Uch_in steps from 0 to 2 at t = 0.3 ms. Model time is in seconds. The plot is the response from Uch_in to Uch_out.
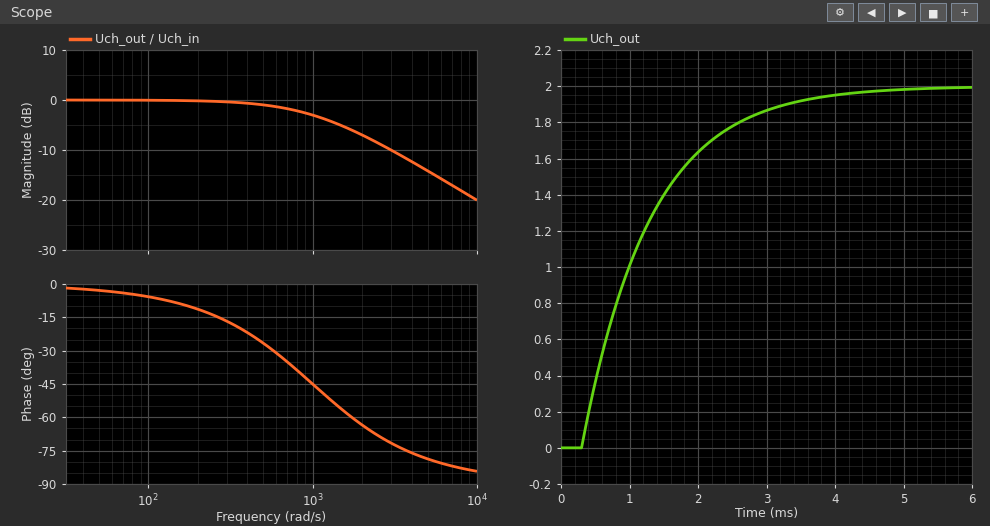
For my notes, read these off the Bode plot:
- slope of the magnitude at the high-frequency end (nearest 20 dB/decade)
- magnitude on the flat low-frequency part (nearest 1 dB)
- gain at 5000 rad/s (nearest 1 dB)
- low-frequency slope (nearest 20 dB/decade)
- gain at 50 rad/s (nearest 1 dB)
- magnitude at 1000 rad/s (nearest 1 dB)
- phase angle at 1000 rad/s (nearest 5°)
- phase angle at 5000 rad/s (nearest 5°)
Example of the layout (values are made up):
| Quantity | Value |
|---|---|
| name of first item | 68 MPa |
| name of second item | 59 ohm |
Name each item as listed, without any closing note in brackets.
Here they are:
| Quantity | Value |
|---|---|
| slope of the magnitude at the high-frequency end | -20 dB/decade |
| magnitude on the flat low-frequency part | 0 dB |
| gain at 5000 rad/s | -14 dB |
| low-frequency slope | 0 dB/decade |
| gain at 50 rad/s | 0 dB |
| magnitude at 1000 rad/s | -3 dB |
| phase angle at 1000 rad/s | -45° |
| phase angle at 5000 rad/s | -80° |
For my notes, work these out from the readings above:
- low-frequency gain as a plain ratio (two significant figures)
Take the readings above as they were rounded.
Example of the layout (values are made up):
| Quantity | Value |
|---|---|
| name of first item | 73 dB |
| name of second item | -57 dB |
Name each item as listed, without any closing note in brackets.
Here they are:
| Quantity | Value |
|---|---|
| low-frequency gain as a plain ratio | 1.0 |
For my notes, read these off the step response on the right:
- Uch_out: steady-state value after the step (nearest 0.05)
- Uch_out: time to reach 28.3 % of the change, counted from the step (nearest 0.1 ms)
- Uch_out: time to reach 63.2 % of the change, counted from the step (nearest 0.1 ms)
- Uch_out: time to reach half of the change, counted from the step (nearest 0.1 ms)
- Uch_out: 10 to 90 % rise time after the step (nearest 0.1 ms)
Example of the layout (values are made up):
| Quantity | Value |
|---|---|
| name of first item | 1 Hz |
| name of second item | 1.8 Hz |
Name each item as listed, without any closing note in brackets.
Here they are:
| Quantity | Value |
|---|---|
| Uch_out: steady-state value after the step | 2.00 |
| Uch_out: time to reach 28.3 % of the change, counted from the step | 0.3 ms |
| Uch_out: time to reach 63.2 % of the change, counted from the step | 1.0 ms |
| Uch_out: time to reach half of the change, counted from the step | 0.7 ms |
| Uch_out: 10 to 90 % rise time after the step | 2.2 ms |
